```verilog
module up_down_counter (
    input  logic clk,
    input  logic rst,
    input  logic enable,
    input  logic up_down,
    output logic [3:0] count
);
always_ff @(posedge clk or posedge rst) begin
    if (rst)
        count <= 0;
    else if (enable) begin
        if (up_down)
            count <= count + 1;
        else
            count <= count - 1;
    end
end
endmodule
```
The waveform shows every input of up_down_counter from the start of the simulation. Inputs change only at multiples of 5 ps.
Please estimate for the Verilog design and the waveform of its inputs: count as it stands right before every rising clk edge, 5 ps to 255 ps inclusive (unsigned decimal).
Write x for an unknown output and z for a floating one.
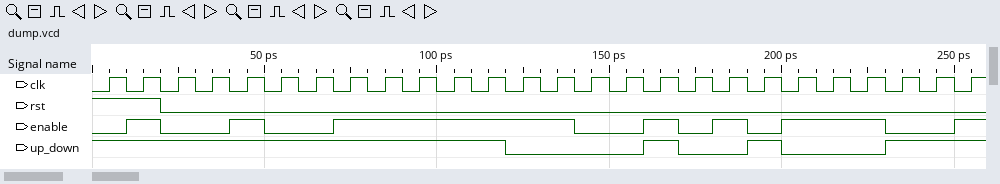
0, 0, 0, 0, 0, 1, 1, 1, 2, 3, 4, 5, 6, 5, 4, 4, 4, 5, 5, 4, 4, 3, 2, 1, 1, 1
